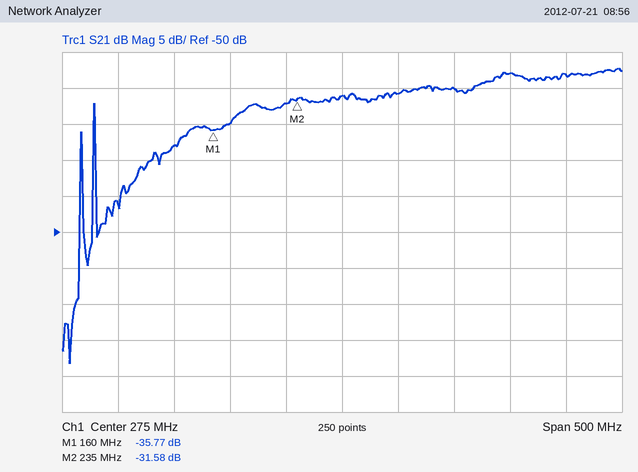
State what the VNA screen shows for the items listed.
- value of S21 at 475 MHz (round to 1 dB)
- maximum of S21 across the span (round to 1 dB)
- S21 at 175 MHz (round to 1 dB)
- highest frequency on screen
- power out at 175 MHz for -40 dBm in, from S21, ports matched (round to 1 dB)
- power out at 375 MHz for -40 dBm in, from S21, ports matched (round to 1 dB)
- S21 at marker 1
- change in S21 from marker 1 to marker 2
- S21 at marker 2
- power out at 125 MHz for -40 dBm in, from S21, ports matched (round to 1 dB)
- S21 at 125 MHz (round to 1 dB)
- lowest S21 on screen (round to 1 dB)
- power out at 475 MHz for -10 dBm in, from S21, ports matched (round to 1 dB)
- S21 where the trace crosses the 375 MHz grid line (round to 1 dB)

-28 dB
-27 dB
-35 dB
525 MHz
-75 dBm
-70 dBm
-35.77 dB
4.19 dB
-31.58 dB
-78 dBm
-38 dB
-68 dB
-38 dBm
-30 dB
